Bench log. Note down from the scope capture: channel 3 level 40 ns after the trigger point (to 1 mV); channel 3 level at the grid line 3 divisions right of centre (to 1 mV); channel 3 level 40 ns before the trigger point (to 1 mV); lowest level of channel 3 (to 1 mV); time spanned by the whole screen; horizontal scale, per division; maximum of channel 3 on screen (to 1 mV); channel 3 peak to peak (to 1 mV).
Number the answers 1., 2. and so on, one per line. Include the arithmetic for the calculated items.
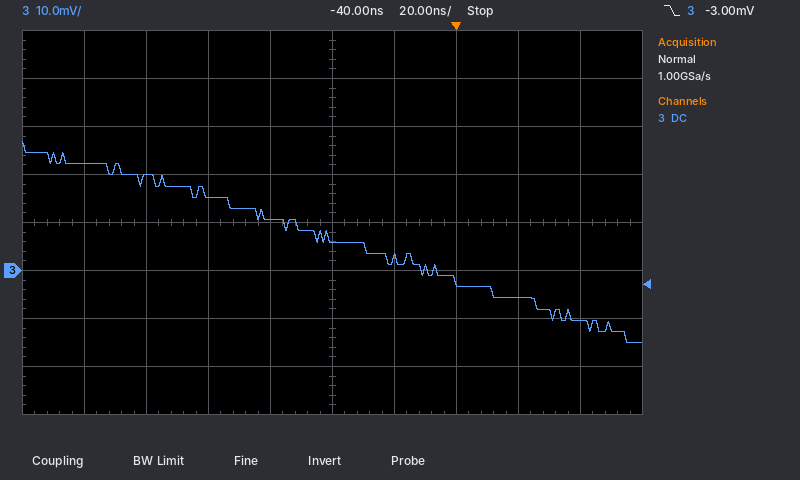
1. -10 mV
2. -6 mV
3. 6 mV
4. -15 mV
5. 200 ns
6. 20 ns
7. 27 mV
8. 27 mV − (-15 mV) = 42 mV
